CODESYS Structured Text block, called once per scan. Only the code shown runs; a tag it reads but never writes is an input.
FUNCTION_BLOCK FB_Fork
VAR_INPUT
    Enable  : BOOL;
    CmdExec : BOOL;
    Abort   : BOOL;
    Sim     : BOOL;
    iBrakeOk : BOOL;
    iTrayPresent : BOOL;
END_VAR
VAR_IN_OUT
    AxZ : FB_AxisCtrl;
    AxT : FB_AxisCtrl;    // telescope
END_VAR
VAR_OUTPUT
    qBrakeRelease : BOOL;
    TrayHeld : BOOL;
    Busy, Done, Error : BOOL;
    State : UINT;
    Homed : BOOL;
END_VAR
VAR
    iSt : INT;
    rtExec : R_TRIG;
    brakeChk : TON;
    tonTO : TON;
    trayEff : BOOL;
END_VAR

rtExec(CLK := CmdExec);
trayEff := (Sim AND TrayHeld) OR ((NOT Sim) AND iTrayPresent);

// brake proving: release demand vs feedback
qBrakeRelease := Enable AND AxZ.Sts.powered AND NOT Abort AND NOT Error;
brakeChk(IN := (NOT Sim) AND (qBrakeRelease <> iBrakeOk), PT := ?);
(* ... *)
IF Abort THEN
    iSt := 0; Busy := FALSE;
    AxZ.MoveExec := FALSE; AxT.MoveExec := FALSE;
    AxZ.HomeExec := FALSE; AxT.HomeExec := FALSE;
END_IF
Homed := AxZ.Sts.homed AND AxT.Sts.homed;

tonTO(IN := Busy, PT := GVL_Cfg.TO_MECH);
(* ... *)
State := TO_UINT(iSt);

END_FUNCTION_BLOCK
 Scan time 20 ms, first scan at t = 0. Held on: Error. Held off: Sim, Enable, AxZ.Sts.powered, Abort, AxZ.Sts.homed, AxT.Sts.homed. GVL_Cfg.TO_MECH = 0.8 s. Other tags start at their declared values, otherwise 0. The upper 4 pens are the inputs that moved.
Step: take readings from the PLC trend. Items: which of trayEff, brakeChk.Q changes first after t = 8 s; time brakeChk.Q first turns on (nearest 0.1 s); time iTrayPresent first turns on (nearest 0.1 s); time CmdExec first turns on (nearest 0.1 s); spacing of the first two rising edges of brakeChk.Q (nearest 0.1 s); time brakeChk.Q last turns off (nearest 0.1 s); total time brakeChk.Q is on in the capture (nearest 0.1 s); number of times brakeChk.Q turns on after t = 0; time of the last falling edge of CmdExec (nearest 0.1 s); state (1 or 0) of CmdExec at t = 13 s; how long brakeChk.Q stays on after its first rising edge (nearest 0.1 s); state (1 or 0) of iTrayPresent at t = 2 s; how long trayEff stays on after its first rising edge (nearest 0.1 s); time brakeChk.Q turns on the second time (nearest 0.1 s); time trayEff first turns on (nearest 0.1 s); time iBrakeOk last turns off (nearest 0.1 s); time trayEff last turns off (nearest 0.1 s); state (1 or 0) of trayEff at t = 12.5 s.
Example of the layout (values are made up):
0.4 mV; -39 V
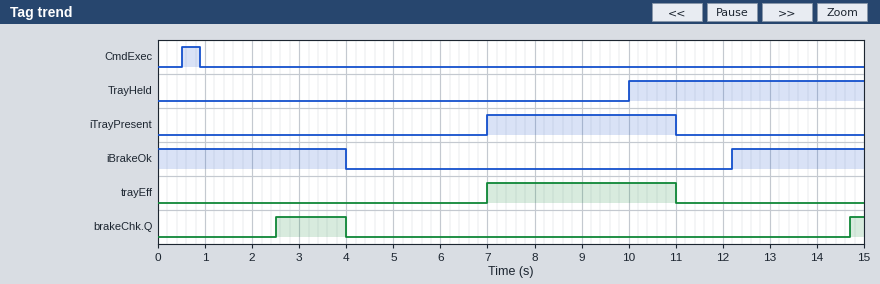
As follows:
trayEff; 2.5 s; 7.0 s; 0.5 s; 12.2 s; 4.0 s; 1.8 s; 2; 0.9 s; 0; 1.5 s; 0; 4.0 s; 14.7 s; 7.0 s; 4.0 s; 11.0 s; 0
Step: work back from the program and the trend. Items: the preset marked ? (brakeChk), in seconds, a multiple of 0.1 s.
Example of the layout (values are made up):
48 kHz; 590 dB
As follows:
2.5 s
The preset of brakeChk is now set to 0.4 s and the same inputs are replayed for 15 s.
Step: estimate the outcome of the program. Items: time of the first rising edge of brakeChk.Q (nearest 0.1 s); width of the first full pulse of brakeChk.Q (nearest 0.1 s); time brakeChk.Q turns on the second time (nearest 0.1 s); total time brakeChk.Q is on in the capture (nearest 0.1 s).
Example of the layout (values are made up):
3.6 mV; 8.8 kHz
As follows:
0.4 s; 3.6 s; 12.6 s; 6.0 s
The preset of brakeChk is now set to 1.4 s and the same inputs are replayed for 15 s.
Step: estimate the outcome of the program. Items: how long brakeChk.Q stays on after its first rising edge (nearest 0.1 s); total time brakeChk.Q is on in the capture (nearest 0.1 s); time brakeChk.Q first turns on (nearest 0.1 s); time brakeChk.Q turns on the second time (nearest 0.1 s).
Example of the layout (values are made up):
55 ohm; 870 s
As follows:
2.6 s; 4.0 s; 1.4 s; 13.6 s
